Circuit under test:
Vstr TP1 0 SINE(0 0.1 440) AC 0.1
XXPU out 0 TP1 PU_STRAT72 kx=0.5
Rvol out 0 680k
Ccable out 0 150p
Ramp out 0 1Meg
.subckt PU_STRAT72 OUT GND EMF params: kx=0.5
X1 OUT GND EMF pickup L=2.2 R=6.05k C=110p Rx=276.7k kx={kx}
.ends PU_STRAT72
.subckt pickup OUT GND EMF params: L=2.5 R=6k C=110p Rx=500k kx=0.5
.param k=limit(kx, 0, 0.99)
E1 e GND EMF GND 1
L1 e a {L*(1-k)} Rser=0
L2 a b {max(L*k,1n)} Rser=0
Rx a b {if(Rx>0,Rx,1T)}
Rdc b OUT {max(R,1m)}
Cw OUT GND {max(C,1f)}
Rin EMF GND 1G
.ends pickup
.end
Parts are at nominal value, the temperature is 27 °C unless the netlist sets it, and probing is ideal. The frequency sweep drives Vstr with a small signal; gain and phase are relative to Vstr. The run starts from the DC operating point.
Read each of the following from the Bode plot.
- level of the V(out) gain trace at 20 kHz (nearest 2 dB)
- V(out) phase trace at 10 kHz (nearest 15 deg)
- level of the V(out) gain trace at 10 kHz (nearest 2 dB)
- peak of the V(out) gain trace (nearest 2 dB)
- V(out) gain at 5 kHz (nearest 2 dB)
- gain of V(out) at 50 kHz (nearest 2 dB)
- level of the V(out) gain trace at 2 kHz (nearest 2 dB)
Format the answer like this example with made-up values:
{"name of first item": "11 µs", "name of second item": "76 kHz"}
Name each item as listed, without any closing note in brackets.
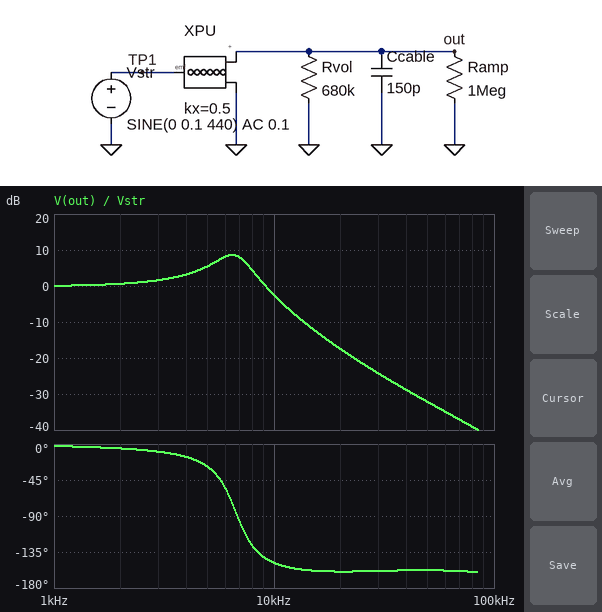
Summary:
{"level of the V(out) gain trace at 20 kHz": "-18 dB", "V(out) phase trace at 10 kHz": "-150 deg", "level of the V(out) gain trace at 10 kHz": "-2 dB", "peak of the V(out) gain trace": "8 dB", "V(out) gain at 5 kHz": "6 dB", "gain of V(out) at 50 kHz": "-32 dB", "level of the V(out) gain trace at 2 kHz": "0 dB"}
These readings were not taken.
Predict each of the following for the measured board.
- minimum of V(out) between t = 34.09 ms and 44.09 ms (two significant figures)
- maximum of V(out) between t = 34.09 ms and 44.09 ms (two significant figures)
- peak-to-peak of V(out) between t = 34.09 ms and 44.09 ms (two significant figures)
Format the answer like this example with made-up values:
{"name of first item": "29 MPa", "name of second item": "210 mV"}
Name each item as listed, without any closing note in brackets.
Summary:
{"minimum of V(out) between t = 34.09 ms and 44.09 ms": "-99 mV", "maximum of V(out) between t = 34.09 ms and 44.09 ms": "99 mV", "peak-to-peak of V(out) between t = 34.09 ms and 44.09 ms": "200 mV"}
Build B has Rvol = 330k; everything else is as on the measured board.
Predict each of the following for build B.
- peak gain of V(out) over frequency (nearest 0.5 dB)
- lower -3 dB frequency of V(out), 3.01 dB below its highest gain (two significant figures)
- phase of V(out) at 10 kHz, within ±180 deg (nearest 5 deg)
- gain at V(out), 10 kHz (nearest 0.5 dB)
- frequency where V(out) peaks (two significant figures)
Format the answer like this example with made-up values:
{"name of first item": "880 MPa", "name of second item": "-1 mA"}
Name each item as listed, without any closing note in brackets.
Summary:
{"peak gain of V(out) over frequency": "6.0 dB", "lower -3 dB frequency of V(out), 3.01 dB below its highest gain": "4.1 kHz", "phase of V(out) at 10 kHz, within ±180 deg": "-140 deg", "gain at V(out), 10 kHz": "-3.0 dB", "frequency where V(out) peaks": "6.3 kHz"}
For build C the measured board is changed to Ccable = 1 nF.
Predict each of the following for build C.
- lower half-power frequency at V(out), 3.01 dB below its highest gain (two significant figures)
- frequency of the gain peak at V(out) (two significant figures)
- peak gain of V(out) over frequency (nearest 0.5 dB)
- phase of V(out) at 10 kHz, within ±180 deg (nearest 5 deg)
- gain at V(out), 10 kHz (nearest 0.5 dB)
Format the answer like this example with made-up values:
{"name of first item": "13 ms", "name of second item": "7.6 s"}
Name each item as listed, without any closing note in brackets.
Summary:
{"lower half-power frequency at V(out), 3.01 dB below its highest gain": "2.7 kHz", "frequency of the gain peak at V(out)": "3.2 kHz", "peak gain of V(out) over frequency": "11.0 dB", "phase of V(out) at 10 kHz, within ±180 deg": "-165 deg", "gain at V(out), 10 kHz": "-18.5 dB"}
